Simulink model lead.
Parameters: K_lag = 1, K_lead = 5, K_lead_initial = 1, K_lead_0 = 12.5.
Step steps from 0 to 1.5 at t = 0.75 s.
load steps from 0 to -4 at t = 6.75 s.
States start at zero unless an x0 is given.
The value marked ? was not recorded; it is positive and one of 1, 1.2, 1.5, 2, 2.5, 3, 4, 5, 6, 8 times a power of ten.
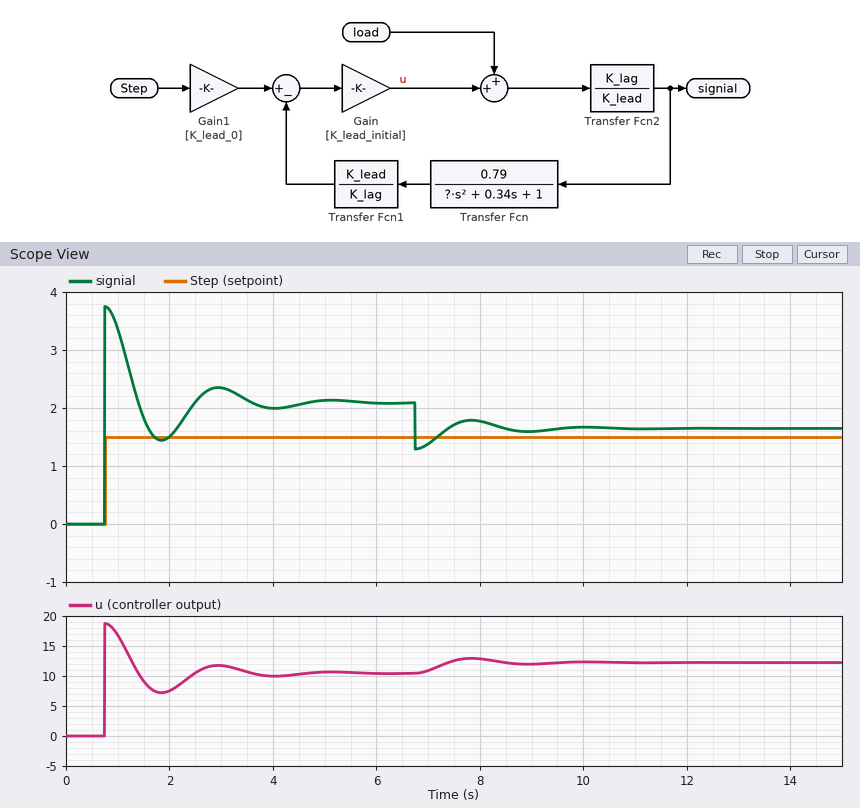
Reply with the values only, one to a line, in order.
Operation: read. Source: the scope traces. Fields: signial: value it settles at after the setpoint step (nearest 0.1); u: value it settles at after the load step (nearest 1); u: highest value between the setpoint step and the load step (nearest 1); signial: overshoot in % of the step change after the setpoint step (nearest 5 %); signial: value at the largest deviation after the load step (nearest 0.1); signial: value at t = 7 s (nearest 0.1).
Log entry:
2.1
12
19
80 %
1.3
1.4
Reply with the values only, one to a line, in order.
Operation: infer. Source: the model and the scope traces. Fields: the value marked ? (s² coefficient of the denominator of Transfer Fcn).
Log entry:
0.2
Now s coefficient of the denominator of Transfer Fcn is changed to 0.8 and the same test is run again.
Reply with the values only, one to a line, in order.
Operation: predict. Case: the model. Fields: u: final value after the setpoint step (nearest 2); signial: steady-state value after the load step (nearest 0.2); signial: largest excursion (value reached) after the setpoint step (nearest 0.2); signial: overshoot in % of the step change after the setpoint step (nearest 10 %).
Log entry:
10
1.6
3.8
80 %
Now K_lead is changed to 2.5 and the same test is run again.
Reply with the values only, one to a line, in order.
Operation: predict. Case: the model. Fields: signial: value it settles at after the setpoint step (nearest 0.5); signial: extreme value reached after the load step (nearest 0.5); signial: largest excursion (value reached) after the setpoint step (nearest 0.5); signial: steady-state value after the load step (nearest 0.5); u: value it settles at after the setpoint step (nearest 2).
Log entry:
4.0
2.5
7.5
3.5
10
